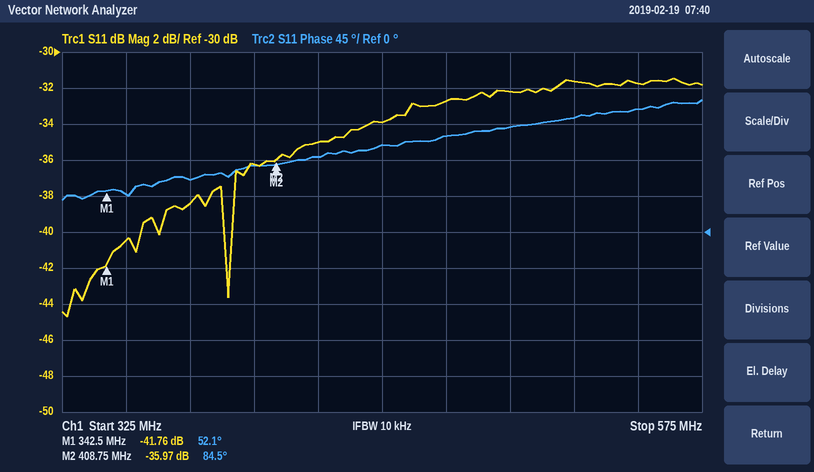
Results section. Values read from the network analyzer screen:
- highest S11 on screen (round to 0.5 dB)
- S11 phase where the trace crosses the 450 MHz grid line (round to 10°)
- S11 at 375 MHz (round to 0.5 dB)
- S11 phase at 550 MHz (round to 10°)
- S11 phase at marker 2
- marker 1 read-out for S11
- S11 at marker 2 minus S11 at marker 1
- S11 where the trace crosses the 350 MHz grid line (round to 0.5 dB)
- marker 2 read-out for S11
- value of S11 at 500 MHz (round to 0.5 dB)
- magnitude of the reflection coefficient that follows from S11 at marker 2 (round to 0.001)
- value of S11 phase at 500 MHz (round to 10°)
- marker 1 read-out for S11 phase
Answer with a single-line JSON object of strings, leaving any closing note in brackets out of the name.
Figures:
{"highest S11 on screen": "-31.5 dB", "S11 phase where the trace crosses the 450 MHz grid line": "110°", "S11 at 375 MHz": "-38.5 dB", "S11 phase at 550 MHz": "150°", "S11 phase at marker 2": "84.5°", "marker 1 read-out for S11": "-41.76 dB", "S11 at marker 2 minus S11 at marker 1": "5.79 dB", "S11 where the trace crosses the 350 MHz grid line": "-40.5 dB", "marker 2 read-out for S11": "-35.97 dB", "value of S11 at 500 MHz": "-32.0 dB", "magnitude of the reflection coefficient that follows from S11 at marker 2": "0.016", "value of S11 phase at 500 MHz": "130°", "marker 1 read-out for S11 phase": "52.1°"}
